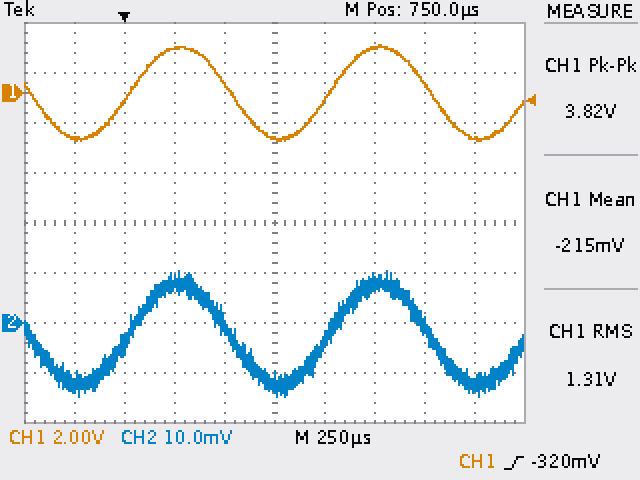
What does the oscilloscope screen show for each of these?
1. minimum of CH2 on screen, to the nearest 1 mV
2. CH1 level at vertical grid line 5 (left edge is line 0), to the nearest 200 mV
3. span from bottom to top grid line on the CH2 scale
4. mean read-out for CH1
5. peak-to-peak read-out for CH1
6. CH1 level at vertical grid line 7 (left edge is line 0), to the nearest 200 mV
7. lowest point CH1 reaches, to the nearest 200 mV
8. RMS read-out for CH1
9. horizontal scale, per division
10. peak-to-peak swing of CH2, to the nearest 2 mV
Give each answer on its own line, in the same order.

-15 mV
-1.8 V
80 mV
-215 mV
3.82 V
1.8 V
-2.0 V
1.31 V
250 µs
26 mV
